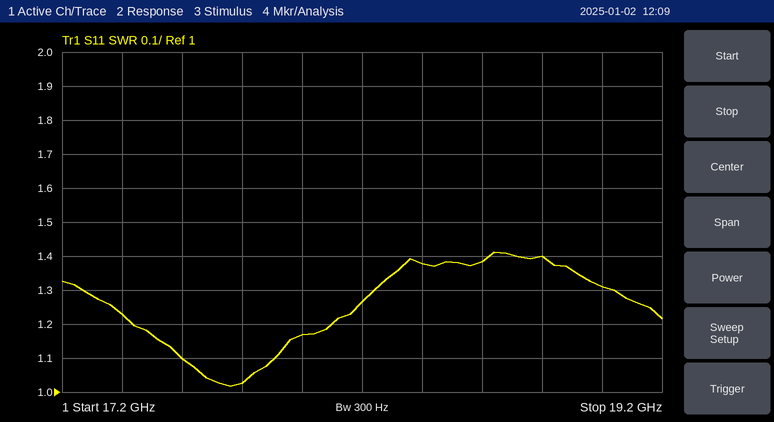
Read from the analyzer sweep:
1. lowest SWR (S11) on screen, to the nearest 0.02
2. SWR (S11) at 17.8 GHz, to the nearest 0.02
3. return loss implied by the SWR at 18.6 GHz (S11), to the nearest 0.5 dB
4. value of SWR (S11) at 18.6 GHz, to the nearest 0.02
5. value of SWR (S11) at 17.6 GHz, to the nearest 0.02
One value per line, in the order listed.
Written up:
1.02
1.02
16.0 dB
1.38
1.10
